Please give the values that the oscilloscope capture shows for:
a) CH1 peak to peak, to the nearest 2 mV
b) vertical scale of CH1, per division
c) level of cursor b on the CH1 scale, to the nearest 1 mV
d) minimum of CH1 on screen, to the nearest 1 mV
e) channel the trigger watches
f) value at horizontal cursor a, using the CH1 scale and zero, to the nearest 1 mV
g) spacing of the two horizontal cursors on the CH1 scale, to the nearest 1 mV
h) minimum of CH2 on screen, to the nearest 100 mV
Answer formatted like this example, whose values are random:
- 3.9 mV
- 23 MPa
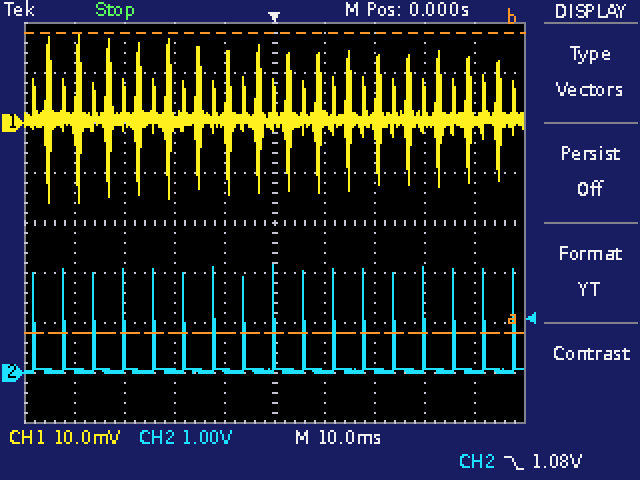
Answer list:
- 34 mV
- 10 mV
- 18 mV
- -16 mV
- CH2
- -42 mV
- 60 mV
- 0.0 V
